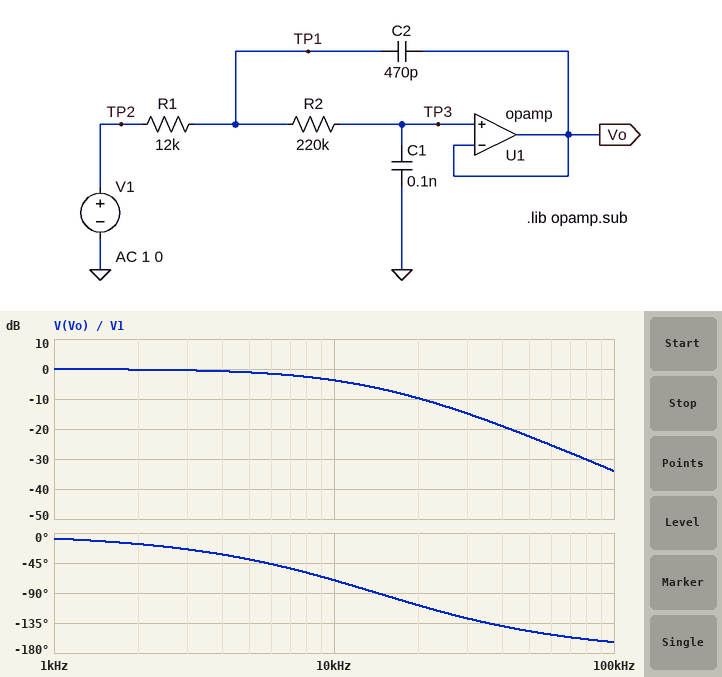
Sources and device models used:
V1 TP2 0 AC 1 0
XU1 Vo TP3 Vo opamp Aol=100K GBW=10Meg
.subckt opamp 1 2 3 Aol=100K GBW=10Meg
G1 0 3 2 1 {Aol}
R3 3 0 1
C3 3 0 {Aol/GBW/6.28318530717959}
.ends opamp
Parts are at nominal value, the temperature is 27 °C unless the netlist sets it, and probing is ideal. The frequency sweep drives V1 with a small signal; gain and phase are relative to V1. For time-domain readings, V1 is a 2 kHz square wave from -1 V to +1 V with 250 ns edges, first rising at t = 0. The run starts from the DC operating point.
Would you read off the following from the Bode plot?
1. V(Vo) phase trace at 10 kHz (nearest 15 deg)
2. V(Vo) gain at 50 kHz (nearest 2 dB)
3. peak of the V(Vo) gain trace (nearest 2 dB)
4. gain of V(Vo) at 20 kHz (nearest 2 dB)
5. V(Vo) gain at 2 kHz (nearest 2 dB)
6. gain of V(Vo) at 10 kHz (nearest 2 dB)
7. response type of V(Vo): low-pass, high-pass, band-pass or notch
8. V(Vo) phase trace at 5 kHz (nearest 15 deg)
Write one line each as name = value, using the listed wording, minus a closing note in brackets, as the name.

V(Vo) phase trace at 10 kHz = -75 deg
V(Vo) gain at 50 kHz = -22 dB
peak of the V(Vo) gain trace = 0 dB
gain of V(Vo) at 20 kHz = -10 dB
V(Vo) gain at 2 kHz = 0 dB
gain of V(Vo) at 10 kHz = -4 dB
response type of V(Vo): low-pass, high-pass, band-pass or notch = low-pass
V(Vo) phase trace at 5 kHz = -45 deg
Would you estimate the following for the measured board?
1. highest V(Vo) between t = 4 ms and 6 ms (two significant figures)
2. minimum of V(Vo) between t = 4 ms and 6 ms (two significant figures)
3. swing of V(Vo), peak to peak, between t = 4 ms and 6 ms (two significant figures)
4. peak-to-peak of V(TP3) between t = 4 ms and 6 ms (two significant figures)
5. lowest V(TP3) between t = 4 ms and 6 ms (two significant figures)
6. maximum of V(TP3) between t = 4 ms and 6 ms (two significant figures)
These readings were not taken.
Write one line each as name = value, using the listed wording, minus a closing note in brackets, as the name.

highest V(Vo) between t = 4 ms and 6 ms = 1.0 V
minimum of V(Vo) between t = 4 ms and 6 ms = -1.0 V
swing of V(Vo), peak to peak, between t = 4 ms and 6 ms = 2.0 V
peak-to-peak of V(TP3) between t = 4 ms and 6 ms = 2.0 V
lowest V(TP3) between t = 4 ms and 6 ms = -1.0 V
maximum of V(TP3) between t = 4 ms and 6 ms = 1.0 V
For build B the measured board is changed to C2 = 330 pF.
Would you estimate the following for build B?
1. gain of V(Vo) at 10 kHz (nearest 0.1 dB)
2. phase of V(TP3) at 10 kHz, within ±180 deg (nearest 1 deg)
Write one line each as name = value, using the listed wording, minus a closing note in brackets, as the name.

gain of V(Vo) at 10 kHz = -4.1 dB
phase of V(TP3) at 10 kHz, within ±180 deg = -66 deg
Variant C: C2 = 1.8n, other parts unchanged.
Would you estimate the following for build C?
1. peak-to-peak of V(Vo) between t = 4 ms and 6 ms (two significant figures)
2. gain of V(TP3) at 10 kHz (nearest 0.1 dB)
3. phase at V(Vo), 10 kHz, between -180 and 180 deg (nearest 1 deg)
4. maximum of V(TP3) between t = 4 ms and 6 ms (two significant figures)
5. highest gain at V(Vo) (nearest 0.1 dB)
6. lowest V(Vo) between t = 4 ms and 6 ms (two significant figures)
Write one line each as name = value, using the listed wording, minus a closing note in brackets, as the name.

peak-to-peak of V(Vo) between t = 4 ms and 6 ms = 2.6 V
gain of V(TP3) at 10 kHz = -4.6 dB
phase at V(Vo), 10 kHz, between -180 and 180 deg = -121 deg
maximum of V(TP3) between t = 4 ms and 6 ms = 1.3 V
highest gain at V(Vo) = 0.9 dB
lowest V(Vo) between t = 4 ms and 6 ms = -1.3 V
